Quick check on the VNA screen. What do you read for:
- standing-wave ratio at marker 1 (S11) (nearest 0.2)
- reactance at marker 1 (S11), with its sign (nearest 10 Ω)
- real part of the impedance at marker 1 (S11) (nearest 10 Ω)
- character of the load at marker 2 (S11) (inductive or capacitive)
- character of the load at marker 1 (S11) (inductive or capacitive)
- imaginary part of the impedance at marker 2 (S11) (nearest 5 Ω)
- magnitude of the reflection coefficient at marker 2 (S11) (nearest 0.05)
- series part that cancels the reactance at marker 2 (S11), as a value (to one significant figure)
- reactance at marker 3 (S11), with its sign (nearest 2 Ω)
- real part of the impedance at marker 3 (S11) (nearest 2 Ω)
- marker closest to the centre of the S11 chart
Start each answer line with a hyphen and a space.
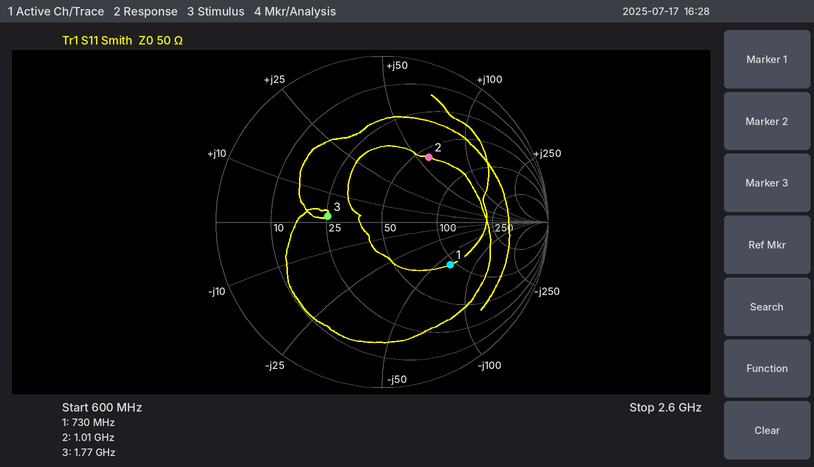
- 2.8
- -60 Ω
- 90 Ω
- inductive
- capacitive
- +60 Ω
- 0.50
- 3 pF
- +2 Ω
- 26 Ω
- marker 3
